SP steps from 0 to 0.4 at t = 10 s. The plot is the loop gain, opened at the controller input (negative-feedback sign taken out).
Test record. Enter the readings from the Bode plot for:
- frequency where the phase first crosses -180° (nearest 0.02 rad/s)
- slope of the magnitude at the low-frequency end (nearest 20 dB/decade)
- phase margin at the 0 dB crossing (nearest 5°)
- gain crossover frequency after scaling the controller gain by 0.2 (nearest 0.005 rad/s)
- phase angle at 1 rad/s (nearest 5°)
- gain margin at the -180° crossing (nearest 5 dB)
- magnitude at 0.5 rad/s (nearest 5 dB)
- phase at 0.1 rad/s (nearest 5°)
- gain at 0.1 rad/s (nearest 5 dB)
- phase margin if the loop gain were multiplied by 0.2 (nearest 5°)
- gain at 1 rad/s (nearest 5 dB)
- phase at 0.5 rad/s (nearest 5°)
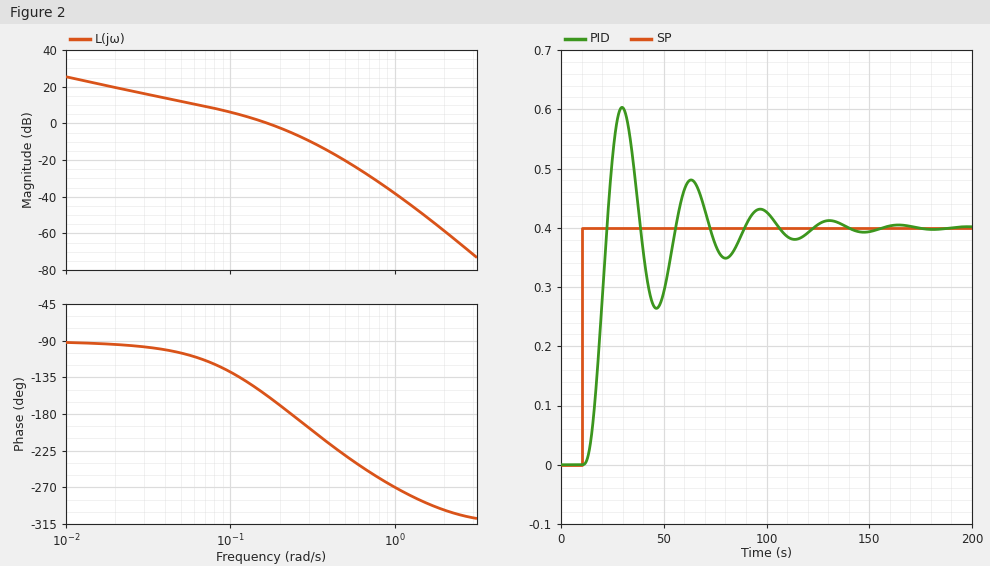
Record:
0.24 rad/s
-20 dB/decade
20°
0.040 rad/s
-270°
5 dB
-20 dB
-130°
5 dB
80°
-40 dB
-230°
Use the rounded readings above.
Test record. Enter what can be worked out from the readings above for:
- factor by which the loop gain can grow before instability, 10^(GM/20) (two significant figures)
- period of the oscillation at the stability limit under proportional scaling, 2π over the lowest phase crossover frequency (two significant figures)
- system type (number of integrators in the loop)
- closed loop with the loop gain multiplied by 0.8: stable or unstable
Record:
1.8
26 s
1
stable
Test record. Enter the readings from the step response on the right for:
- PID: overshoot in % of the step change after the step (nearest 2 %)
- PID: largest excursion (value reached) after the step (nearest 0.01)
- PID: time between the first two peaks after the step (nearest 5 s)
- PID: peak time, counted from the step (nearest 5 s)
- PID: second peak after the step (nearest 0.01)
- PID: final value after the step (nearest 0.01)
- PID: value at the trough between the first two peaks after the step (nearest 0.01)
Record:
50 %
0.60
35 s
20 s
0.48
0.40
0.26
